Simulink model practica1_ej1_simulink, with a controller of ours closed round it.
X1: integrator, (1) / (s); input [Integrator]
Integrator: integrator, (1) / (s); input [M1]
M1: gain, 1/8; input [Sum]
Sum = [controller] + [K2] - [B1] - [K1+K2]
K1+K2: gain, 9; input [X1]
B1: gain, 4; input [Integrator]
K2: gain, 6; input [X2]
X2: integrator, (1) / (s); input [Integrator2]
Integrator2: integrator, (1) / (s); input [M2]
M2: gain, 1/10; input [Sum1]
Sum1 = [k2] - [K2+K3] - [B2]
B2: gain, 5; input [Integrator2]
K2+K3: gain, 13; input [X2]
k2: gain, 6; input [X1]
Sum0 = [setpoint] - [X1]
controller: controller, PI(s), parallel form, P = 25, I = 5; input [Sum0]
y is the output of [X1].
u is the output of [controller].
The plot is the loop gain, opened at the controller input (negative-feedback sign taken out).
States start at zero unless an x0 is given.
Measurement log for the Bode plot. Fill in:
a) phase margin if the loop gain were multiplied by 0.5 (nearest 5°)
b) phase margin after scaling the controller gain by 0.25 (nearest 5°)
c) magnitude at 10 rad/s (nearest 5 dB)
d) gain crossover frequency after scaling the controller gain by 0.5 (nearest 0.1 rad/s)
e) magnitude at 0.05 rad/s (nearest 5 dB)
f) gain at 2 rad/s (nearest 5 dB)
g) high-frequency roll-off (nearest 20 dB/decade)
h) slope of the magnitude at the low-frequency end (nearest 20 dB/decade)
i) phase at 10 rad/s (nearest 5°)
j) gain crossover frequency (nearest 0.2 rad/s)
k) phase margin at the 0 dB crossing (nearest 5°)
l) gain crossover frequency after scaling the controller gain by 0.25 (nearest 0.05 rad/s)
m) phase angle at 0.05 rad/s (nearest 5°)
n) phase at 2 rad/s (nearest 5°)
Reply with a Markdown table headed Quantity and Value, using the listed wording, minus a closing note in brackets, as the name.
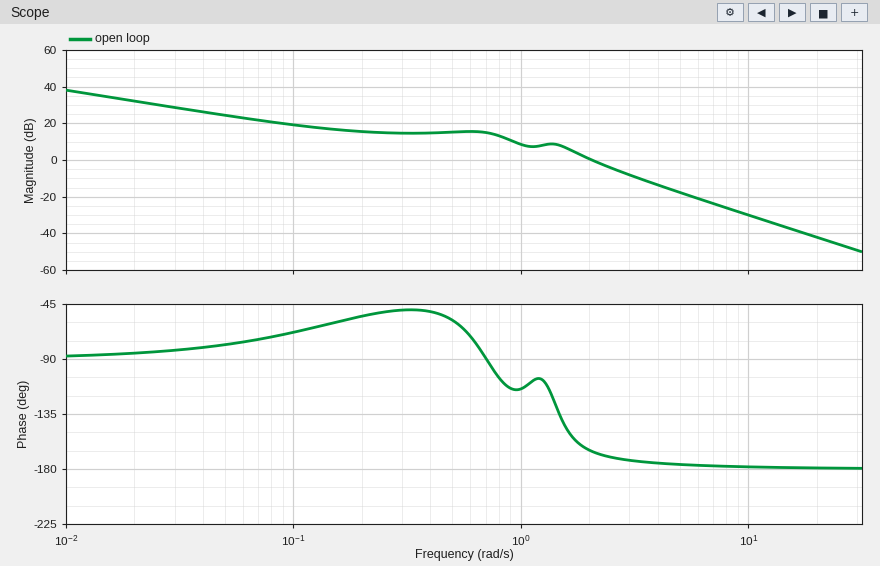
| Quantity | Value |
|---|---|
| phase margin if the loop gain were multiplied by 0.5 | 30° |
| phase margin after scaling the controller gain by 0.25 | 70° |
| magnitude at 10 rad/s | -30 dB |
| gain crossover frequency after scaling the controller gain by 0.5 | 1.6 rad/s |
| magnitude at 0.05 rad/s | 25 dB |
| gain at 2 rad/s | 0 dB |
| high-frequency roll-off | -40 dB/decade |
| slope of the magnitude at the low-frequency end | -20 dB/decade |
| phase at 10 rad/s | -180° |
| gain crossover frequency | 2.0 rad/s |
| phase margin at the 0 dB crossing | 15° |
| gain crossover frequency after scaling the controller gain by 0.25 | 0.85 rad/s |
| phase angle at 0.05 rad/s | -80° |
| phase at 2 rad/s | -165° |
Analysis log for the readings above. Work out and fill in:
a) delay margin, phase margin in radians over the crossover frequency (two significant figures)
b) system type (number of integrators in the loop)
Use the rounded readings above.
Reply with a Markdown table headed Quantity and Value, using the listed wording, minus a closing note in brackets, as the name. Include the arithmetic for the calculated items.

| Quantity | Value |
|---|---|
| delay margin, phase margin in radians over the crossover frequency | 15 × π / 180 / 2 = 0.13 s |
| system type | 1 |
